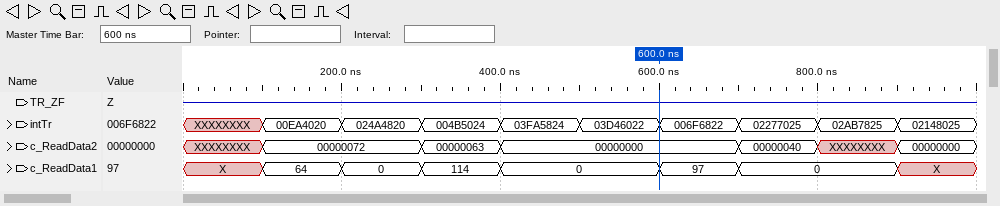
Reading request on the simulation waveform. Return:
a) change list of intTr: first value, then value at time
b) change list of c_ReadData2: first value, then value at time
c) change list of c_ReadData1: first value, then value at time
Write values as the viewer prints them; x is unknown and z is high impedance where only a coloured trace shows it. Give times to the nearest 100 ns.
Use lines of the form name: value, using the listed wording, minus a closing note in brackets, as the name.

change list of intTr: first value, then value at time: XXXXXXXX, 00EA4020 at 100 ns, 024A4820 at 200 ns, 004B5024 at 300 ns, 03FA5824 at 400 ns, 03D46022 at 500 ns, 006F6822 at 600 ns, 02277025 at 700 ns, 02AB7825 at 800 ns, 02148025 at 900 ns
change list of c_ReadData2: first value, then value at time: XXXXXXXX, 00000072 at 100 ns, 00000063 at 300 ns, 00000000 at 400 ns, 00000040 at 700 ns, XXXXXXXX at 800 ns, 00000000 at 900 ns
change list of c_ReadData1: first value, then value at time: X, 64 at 100 ns, 0 at 200 ns, 114 at 300 ns, 0 at 400 ns, 97 at 600 ns, 0 at 700 ns, X at 900 ns
